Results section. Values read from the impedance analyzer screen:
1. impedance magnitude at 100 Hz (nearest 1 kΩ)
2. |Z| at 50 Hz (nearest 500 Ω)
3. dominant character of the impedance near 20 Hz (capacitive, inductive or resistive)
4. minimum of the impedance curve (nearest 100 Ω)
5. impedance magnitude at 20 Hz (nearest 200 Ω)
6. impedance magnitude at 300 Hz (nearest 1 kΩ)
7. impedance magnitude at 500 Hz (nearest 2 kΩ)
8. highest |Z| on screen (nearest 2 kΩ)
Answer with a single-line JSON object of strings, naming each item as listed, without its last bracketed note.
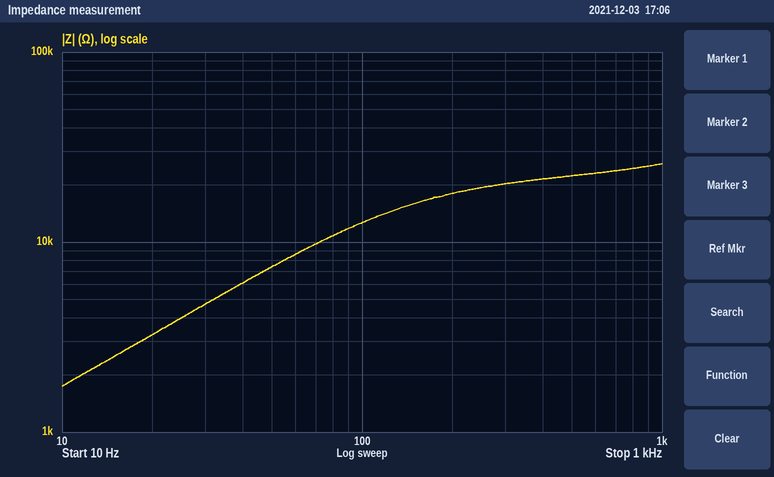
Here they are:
{"impedance magnitude at 100 Hz": "13 kΩ", "|Z| at 50 Hz": "7.5 kΩ", "dominant character of the impedance near 20 Hz": "inductive", "minimum of the impedance curve": "1.7 kΩ", "impedance magnitude at 20 Hz": "3.2 kΩ", "impedance magnitude at 300 Hz": "20 kΩ", "impedance magnitude at 500 Hz": "22 kΩ", "highest |Z| on screen": "26 kΩ"}
